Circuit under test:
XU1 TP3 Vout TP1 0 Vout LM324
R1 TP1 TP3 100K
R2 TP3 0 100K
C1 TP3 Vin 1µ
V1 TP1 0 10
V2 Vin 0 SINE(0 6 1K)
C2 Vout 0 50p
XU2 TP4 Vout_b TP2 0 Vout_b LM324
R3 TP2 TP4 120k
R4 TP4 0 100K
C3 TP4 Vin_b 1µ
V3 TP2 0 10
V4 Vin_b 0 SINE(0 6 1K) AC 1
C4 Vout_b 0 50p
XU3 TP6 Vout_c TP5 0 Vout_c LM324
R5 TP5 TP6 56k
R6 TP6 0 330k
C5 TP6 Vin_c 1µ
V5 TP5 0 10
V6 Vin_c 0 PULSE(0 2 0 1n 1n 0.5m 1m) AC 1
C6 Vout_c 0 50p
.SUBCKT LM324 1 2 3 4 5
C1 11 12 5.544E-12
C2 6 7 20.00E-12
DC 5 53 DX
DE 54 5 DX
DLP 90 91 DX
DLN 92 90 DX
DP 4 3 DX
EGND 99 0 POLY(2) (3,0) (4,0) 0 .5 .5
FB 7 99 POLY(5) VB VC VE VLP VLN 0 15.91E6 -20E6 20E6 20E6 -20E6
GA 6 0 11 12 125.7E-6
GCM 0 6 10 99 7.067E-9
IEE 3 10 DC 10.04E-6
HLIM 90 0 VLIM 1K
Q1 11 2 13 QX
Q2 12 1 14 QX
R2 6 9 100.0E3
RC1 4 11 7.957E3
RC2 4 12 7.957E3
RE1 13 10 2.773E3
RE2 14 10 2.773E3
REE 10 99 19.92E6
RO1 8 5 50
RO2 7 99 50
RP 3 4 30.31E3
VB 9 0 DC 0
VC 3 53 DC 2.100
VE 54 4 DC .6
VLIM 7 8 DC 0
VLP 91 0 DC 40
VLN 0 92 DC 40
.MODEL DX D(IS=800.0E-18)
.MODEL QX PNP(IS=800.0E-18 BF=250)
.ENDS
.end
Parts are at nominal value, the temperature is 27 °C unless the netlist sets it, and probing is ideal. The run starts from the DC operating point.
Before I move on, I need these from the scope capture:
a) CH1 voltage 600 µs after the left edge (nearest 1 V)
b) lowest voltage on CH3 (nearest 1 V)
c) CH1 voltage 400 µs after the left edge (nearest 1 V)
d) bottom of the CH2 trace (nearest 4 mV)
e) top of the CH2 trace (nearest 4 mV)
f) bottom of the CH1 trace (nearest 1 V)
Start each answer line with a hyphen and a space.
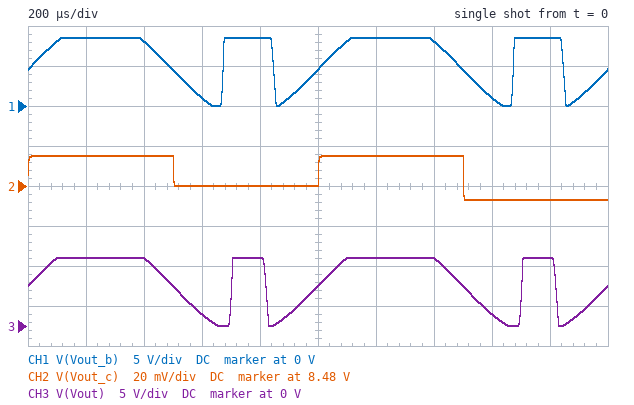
- 1 V
- 0 V
- 8 V
- 8.472 V
- 8.496 V
- 0 V
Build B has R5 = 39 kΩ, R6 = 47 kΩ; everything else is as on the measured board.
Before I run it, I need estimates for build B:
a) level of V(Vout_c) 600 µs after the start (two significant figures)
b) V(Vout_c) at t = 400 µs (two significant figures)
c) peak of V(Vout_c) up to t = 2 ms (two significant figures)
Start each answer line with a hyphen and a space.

- 5.4 V
- 7.4 V
- 7.5 V
